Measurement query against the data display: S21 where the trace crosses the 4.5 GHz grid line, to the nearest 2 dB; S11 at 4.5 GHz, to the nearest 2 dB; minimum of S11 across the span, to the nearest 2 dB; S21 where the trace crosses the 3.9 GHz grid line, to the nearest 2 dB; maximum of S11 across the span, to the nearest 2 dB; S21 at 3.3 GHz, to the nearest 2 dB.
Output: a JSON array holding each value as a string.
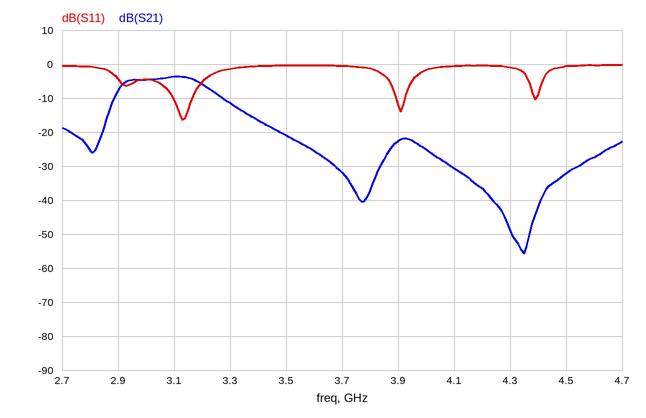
["-32 dB", "0 dB", "-16 dB", "-22 dB", "0 dB", "-12 dB"]
